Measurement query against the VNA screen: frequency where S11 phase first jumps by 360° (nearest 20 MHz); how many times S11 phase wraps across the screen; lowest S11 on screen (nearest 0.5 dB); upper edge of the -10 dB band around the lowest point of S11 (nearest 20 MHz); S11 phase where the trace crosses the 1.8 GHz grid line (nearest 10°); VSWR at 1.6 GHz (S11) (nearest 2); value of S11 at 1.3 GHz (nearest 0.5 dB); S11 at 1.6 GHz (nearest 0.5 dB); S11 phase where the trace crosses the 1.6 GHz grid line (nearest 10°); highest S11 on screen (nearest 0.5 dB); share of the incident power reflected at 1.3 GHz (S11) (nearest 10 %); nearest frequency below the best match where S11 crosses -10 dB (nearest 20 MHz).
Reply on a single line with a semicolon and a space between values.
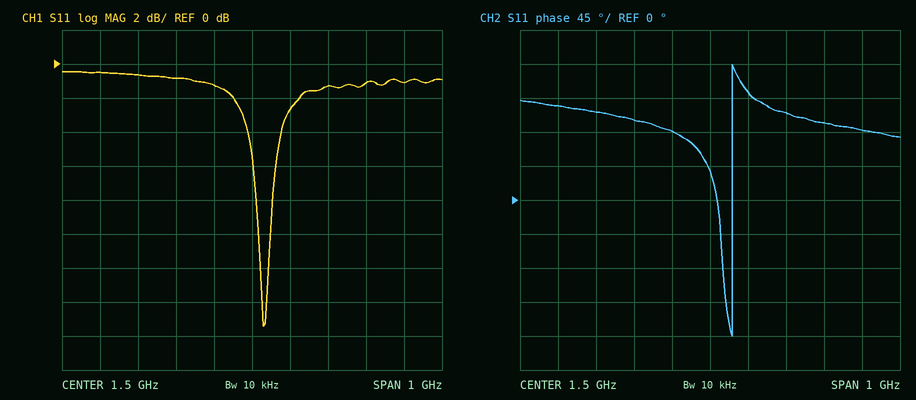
1.56 GHz; 1; -15.5 dB; 1.54 GHz; 100°; 6; -1.0 dB; -2.5 dB; 140°; -0.5 dB; 80 %; 1.52 GHz
